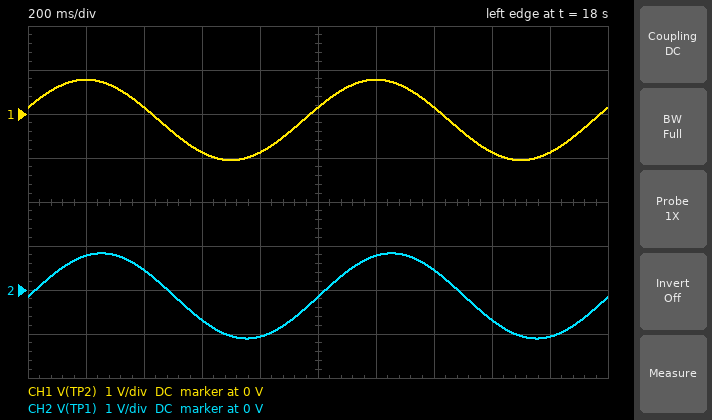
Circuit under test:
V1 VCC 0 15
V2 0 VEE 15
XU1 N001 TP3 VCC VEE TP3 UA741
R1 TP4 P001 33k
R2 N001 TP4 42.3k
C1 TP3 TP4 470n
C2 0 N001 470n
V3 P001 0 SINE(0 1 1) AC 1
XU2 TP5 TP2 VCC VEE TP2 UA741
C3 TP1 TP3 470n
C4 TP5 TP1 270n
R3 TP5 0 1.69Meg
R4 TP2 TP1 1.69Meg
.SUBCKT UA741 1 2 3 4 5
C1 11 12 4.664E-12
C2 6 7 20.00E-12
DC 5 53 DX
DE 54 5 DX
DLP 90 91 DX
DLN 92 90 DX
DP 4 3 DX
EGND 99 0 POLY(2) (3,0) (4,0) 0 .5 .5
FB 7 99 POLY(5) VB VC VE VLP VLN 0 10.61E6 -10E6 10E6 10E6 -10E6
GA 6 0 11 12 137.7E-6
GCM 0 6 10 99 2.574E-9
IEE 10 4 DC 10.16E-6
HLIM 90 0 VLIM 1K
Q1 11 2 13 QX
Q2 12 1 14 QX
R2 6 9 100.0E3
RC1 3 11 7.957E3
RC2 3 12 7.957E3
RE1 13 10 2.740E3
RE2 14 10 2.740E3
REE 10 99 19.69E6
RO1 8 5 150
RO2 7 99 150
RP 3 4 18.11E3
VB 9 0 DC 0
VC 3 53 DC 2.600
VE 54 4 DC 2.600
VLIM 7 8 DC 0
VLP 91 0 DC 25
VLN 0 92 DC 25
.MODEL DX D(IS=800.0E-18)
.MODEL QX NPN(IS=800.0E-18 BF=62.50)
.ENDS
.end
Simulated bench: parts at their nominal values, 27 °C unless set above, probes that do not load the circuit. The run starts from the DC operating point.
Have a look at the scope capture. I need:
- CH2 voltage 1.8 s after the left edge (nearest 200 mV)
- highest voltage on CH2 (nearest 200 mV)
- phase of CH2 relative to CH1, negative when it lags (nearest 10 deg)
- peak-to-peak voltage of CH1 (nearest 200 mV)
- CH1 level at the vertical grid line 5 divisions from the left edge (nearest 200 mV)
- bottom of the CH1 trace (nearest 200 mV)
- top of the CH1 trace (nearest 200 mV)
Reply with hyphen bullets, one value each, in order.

- -1.0 V
- 800 mV
- -20 deg
- 1.8 V
- 200 mV
- -1.0 V
- 800 mV
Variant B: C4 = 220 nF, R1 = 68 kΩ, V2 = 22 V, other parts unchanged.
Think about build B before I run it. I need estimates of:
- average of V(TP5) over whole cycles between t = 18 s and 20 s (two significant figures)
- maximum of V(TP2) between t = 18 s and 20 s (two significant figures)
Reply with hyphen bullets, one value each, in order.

- -140 mV
- 740 mV
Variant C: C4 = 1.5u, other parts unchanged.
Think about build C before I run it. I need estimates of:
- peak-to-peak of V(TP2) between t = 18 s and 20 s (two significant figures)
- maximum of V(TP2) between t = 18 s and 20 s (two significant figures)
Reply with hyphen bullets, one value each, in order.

- 1.9 V
- 830 mV
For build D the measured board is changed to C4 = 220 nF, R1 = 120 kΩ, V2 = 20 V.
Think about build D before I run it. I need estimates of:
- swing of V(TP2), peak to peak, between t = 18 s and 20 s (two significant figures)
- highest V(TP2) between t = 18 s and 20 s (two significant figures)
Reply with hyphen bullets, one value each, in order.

- 1.7 V
- 710 mV
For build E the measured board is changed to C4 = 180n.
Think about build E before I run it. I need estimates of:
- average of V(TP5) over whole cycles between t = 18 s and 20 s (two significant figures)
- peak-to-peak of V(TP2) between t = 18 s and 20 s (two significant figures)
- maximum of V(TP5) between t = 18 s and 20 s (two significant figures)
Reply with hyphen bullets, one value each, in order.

- -130 mV
- 1.7 V
- 720 mV
